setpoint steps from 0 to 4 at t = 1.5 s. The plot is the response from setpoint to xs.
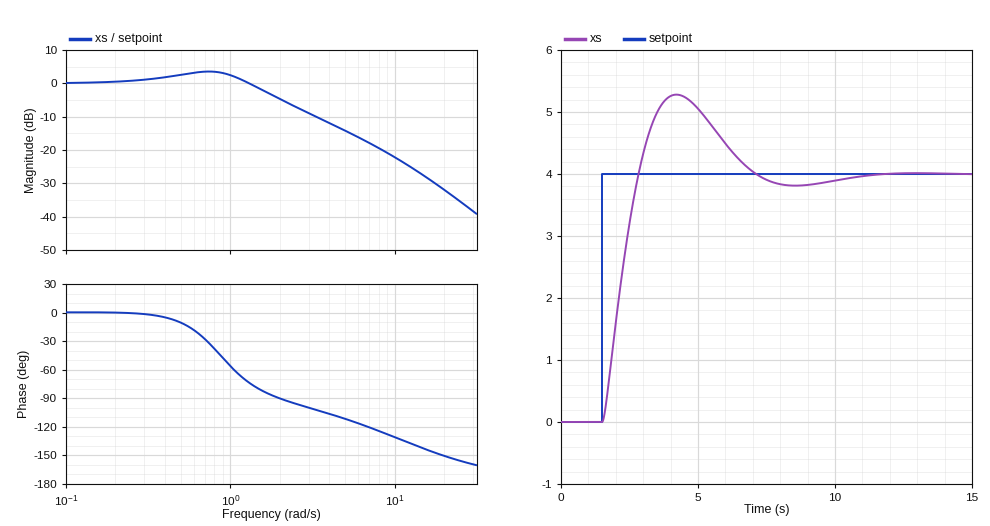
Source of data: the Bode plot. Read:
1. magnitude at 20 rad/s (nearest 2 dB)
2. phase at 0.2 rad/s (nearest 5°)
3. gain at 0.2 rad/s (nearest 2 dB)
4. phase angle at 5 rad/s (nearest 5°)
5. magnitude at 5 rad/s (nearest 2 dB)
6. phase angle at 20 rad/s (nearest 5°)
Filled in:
-32 dB
0°
0 dB
-110°
-14 dB
-150°
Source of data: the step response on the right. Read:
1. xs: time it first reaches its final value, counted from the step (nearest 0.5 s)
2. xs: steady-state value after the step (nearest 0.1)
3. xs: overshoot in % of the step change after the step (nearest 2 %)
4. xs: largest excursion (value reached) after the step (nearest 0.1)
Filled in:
1.5 s
4.0
32 %
5.3
